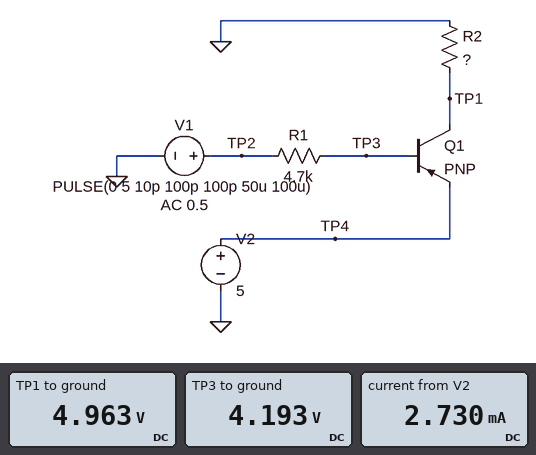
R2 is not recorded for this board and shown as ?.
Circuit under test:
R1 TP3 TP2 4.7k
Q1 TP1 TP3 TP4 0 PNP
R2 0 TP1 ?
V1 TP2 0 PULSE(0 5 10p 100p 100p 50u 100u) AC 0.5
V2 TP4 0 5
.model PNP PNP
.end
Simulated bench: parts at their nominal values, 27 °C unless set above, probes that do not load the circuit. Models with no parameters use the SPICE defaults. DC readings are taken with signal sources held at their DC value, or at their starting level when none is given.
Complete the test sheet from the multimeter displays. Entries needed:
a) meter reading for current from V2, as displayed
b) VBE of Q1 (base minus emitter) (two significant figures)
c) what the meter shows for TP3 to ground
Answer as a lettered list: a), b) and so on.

a) 2.730 mA
b) -810 mV
c) 4.193 V
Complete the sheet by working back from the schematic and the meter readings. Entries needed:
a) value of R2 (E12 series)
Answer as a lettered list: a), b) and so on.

a) 2.7 kΩ
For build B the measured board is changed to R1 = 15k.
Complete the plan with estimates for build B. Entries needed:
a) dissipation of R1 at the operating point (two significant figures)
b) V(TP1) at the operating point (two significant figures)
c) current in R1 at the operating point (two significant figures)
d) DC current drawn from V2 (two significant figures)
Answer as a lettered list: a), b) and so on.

a) 1.2 mW
b) 4.9 V
c) 280 µA
d) 2.1 mA
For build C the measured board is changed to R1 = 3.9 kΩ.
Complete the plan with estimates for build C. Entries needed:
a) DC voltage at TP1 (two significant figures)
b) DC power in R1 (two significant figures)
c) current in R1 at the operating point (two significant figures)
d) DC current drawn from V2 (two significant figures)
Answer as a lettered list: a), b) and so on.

a) 5.0 V
b) 4.5 mW
c) 1.1 mA
d) 2.9 mA
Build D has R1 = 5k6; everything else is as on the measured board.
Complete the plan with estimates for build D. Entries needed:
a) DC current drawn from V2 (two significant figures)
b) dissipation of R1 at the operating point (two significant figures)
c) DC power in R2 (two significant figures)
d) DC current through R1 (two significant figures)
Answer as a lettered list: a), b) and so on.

a) 2.6 mA
b) 3.1 mW
c) 9.1 mW
d) 750 µA
